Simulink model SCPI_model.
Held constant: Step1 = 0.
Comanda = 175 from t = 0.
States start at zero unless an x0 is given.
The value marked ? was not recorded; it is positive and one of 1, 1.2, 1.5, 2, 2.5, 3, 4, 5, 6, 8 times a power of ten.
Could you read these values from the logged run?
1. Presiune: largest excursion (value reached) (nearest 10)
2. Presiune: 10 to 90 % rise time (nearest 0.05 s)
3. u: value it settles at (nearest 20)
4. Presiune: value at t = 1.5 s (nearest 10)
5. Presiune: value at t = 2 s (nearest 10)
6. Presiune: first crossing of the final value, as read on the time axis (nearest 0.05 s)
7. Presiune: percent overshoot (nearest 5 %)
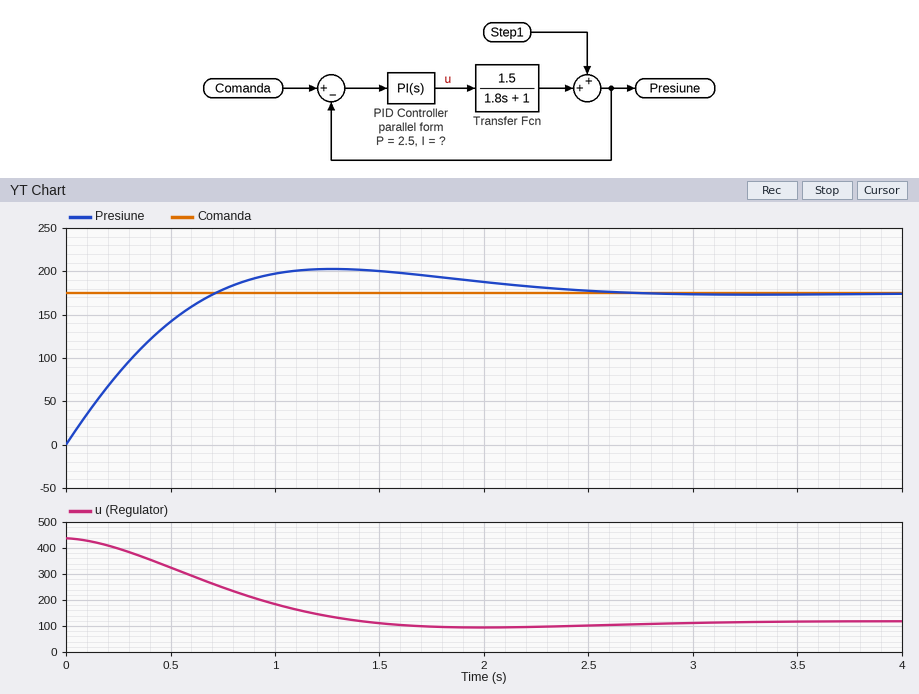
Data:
200
0.55 s
120
200
190
0.70 s
15 %
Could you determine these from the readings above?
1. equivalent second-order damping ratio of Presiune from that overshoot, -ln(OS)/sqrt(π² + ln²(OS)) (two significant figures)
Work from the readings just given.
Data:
0.52
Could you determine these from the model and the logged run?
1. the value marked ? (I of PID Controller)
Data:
5
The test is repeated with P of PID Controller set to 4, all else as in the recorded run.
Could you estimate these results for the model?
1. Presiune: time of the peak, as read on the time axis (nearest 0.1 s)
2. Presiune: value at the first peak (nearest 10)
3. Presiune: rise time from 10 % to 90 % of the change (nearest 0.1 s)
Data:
1.2 s
190
0.5 s
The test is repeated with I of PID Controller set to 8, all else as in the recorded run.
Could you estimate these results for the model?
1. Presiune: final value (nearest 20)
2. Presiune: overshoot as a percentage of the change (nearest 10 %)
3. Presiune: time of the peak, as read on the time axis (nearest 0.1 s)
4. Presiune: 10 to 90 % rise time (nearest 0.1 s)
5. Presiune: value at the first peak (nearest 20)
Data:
180
20 %
1.0 s
0.4 s
220
